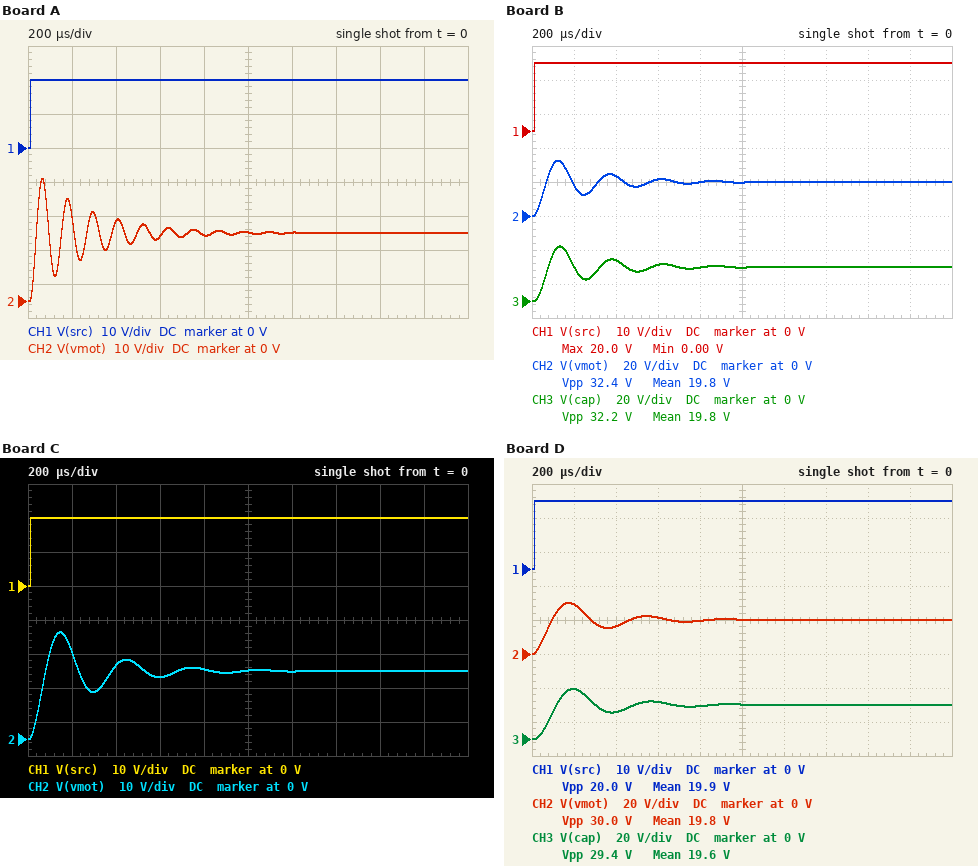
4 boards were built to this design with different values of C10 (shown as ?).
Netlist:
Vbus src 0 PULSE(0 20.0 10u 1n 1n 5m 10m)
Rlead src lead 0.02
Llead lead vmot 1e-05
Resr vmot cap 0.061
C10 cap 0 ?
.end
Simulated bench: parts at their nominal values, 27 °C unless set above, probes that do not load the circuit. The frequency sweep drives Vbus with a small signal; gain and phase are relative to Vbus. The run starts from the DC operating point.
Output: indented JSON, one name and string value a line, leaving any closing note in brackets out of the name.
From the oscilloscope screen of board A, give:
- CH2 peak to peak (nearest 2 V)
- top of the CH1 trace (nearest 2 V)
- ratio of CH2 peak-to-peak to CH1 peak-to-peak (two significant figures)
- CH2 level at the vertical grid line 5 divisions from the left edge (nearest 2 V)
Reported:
{
  "CH2 peak to peak": "36 V",
  "top of the CH1 trace": "20 V",
  "ratio of CH2 peak-to-peak to CH1 peak-to-peak": "1.8",
  "CH2 level at the vertical grid line 5 divisions from the left edge": "20 V"
}
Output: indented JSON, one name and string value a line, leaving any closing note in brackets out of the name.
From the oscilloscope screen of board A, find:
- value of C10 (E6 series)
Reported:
{
  "value of C10": "33 µF"
}
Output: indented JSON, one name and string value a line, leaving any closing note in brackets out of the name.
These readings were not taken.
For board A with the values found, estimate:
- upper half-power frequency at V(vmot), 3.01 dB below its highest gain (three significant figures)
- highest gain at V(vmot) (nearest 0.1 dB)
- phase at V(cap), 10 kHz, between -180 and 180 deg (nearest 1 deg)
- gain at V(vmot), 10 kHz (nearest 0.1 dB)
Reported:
{
  "upper half-power frequency at V(vmot), 3.01 dB below its highest gain": "9.34 kHz",
  "highest gain at V(vmot)": "16.7 dB",
  "phase at V(cap), 10 kHz, between -180 and 180 deg": "-151 deg",
  "gain at V(vmot), 10 kHz": "9.3 dB"
}
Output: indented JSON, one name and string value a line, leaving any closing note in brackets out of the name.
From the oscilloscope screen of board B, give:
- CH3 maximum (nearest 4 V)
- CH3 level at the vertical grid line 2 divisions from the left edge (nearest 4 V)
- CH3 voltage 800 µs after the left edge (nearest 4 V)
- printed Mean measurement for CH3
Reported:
{
  "CH3 maximum": "32 V",
  "CH3 level at the vertical grid line 2 divisions from the left edge": "24 V",
  "CH3 voltage 800 µs after the left edge": "20 V",
  "printed Mean measurement for CH3": "19.8 V"
}
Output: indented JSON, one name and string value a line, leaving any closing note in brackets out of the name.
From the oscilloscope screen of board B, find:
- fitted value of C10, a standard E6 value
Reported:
{
  "fitted value of C10, a standard E6 value": "150 µF"
}
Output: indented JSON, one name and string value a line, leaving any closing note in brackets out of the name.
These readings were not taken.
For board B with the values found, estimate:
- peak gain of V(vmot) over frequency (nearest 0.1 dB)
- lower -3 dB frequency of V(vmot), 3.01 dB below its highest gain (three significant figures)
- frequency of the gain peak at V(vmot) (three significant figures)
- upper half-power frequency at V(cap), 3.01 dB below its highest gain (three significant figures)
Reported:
{
  "peak gain of V(vmot) over frequency": "10.4 dB",
  "lower -3 dB frequency of V(vmot), 3.01 dB below its highest gain": "3.30 kHz",
  "frequency of the gain peak at V(vmot)": "4.01 kHz",
  "upper half-power frequency at V(cap), 3.01 dB below its highest gain": "4.61 kHz"
}
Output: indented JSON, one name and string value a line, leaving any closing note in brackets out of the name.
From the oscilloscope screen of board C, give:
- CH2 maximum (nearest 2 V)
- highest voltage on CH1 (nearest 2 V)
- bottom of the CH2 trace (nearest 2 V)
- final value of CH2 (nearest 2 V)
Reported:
{
  "CH2 maximum": "32 V",
  "highest voltage on CH1": "20 V",
  "bottom of the CH2 trace": "0 V",
  "final value of CH2": "20 V"
}
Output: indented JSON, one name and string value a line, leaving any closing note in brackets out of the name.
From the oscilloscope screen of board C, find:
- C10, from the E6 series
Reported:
{
  "C10, from the E6 series": "220 µF"
}
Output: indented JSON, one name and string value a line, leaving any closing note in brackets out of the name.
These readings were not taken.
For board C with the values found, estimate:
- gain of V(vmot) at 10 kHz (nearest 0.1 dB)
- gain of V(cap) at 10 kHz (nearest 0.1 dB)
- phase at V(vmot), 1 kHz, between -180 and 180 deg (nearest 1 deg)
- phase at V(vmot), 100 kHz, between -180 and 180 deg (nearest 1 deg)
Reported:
{
  "gain of V(vmot) at 10 kHz": "-15.5 dB",
  "gain of V(cap) at 10 kHz": "-17.8 dB",
  "phase at V(vmot), 1 kHz, between -180 and 180 deg": "-2 deg",
  "phase at V(vmot), 100 kHz, between -180 and 180 deg": "-96 deg"
}
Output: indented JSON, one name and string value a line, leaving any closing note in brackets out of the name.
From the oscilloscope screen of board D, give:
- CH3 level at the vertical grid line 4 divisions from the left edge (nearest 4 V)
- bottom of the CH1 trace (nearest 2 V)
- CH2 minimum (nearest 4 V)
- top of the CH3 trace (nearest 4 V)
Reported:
{
  "CH3 level at the vertical grid line 4 divisions from the left edge": "20 V",
  "bottom of the CH1 trace": "0 V",
  "CH2 minimum": "0 V",
  "top of the CH3 trace": "28 V"
}
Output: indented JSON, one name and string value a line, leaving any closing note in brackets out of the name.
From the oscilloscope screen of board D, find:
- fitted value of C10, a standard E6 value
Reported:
{
  "fitted value of C10, a standard E6 value": "330 µF"
}
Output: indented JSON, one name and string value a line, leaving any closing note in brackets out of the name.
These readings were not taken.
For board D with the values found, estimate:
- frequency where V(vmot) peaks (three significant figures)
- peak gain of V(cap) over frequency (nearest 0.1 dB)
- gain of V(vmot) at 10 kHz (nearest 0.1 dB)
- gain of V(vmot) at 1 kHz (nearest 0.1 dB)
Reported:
{
  "frequency where V(vmot) peaks": "2.63 kHz",
  "peak gain of V(cap) over frequency": "6.9 dB",
  "gain of V(vmot) at 10 kHz": "-17.5 dB",
  "gain of V(vmot) at 1 kHz": "1.1 dB"
}
